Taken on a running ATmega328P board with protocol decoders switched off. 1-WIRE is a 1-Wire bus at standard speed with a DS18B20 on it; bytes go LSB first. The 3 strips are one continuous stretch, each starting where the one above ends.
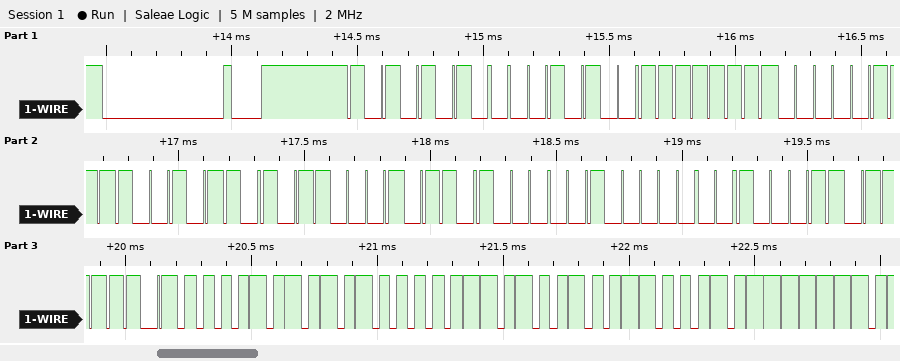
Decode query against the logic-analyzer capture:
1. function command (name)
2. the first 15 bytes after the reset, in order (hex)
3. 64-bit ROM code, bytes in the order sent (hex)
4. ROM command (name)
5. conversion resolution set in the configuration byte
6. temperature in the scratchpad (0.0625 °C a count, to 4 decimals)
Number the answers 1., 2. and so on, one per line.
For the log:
1. Read Scratchpad
2. 55 28 FF E0 69 8D 16 04 C4 BE 50 05 4B 46 7F
3. 28 FF E0 69 8D 16 04 C4
4. Match ROM
5. 12 bits
6. 85.0000 °C
